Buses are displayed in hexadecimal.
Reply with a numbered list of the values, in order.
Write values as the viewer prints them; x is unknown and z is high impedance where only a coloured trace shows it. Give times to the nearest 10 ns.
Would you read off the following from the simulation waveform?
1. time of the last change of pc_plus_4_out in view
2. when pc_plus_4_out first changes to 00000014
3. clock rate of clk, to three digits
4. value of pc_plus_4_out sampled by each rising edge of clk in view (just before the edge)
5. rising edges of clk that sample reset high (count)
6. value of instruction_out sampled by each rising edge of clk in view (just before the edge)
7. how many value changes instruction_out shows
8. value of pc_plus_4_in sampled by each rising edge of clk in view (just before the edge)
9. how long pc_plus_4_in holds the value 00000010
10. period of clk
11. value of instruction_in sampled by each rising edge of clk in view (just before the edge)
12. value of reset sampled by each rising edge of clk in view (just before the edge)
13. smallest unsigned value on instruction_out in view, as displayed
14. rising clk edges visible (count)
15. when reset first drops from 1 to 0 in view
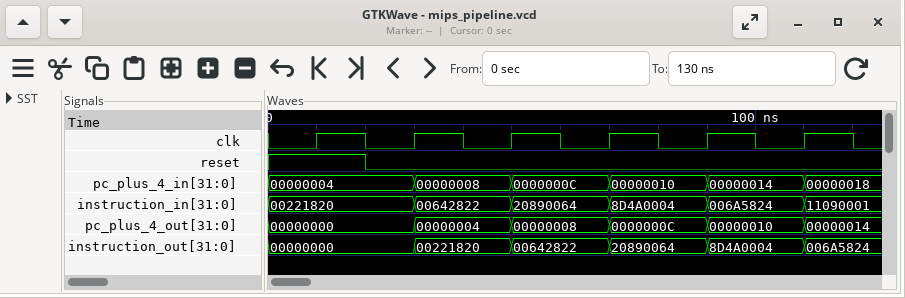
1. 110 ns
2. 110 ns
3. 50.0 MHz
4. 00000000, 00000000, 00000004, 00000008, 0000000C, 00000010
5. 1
6. 00000000, 00000000, 00221820, 00642822, 20890064, 8D4A0004
7. 5
8. 00000004, 00000004, 00000008, 0000000C, 00000010, 00000014
9. 20 ns
10. 20 ns
11. 00221820, 00221820, 00642822, 20890064, 8D4A0004, 006A5824
12. 1 0 0 0 0 0
13. 00000000
14. 6
15. 20 ns
